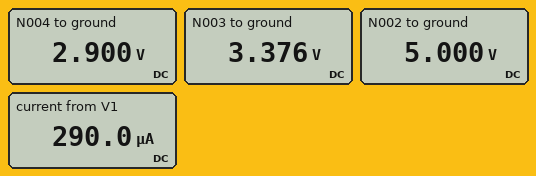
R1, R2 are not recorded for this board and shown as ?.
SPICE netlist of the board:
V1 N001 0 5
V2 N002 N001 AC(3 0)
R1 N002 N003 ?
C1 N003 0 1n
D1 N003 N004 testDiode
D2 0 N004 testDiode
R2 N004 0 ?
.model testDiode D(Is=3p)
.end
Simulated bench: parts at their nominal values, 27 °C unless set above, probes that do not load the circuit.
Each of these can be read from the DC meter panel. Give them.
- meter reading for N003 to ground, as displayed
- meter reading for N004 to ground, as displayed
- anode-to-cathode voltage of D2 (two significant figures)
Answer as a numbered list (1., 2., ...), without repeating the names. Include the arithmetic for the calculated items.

1. 3.376 V
2. 2.900 V
3. 0 V - 2.9 V = -2.9 V
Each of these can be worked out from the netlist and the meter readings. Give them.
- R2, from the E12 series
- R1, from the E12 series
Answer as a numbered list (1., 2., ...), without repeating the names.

1. 10 kΩ
2. 5.6 kΩ
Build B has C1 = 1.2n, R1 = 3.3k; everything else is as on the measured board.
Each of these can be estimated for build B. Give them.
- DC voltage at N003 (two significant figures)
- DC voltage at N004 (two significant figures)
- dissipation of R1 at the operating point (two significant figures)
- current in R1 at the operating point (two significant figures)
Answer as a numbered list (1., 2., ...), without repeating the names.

1. 3.9 V
2. 3.4 V
3. 380 µW
4. 340 µA
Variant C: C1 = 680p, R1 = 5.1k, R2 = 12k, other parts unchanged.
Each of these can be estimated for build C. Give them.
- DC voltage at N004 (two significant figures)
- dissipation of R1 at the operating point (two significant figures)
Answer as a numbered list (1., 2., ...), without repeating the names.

1. 3.2 V
2. 360 µW
